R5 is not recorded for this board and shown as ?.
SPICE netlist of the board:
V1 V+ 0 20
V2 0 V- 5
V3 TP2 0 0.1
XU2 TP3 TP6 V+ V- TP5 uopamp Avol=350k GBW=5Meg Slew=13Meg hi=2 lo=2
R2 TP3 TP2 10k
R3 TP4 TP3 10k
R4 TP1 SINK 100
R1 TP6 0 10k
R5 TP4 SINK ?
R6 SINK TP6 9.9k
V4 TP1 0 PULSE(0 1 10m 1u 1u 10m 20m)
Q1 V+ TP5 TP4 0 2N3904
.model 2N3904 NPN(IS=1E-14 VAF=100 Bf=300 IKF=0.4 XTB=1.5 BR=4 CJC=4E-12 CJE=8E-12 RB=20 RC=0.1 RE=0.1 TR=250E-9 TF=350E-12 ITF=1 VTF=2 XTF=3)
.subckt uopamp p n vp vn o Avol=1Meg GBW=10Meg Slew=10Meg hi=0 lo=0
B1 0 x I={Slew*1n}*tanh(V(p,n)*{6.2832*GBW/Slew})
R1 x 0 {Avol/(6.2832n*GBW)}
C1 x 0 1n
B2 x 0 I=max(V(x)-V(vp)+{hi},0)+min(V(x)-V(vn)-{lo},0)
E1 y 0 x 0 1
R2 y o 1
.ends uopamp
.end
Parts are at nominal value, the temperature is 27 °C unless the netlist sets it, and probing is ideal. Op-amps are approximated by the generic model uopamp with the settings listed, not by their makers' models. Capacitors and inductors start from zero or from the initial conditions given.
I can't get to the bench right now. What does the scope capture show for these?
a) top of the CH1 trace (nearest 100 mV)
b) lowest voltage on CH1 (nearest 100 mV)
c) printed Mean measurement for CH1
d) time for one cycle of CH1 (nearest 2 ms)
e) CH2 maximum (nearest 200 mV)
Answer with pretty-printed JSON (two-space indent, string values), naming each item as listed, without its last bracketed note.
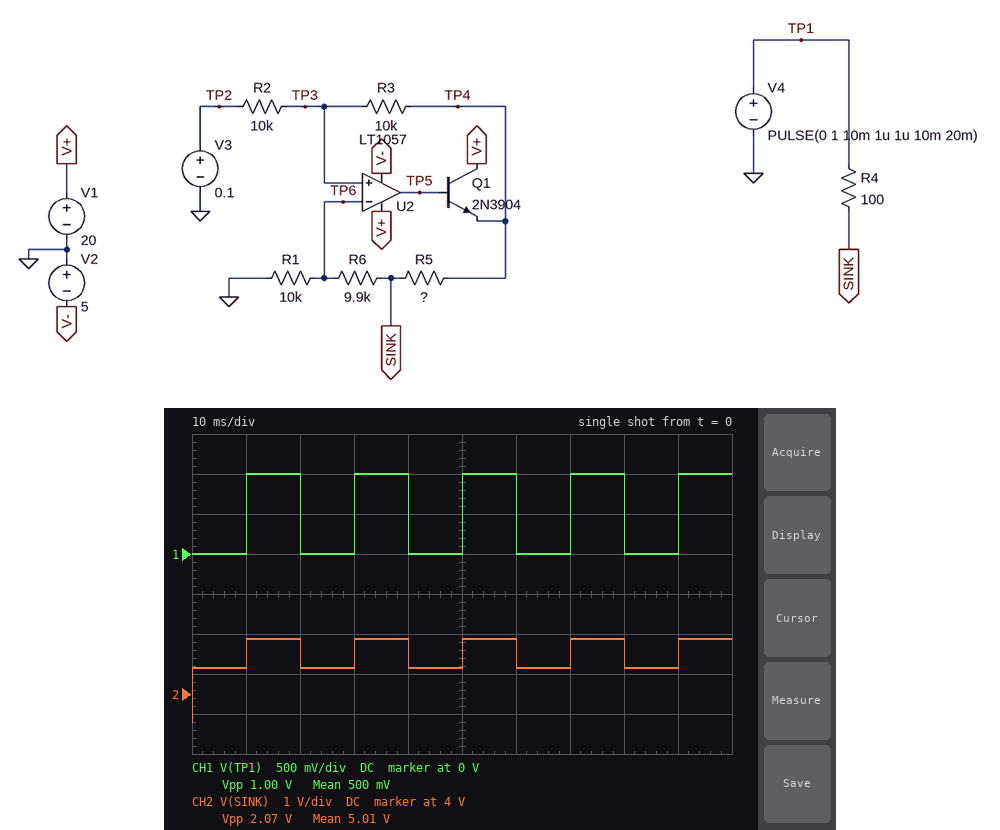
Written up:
{
  "top of the CH1 trace": "1.0 V",
  "lowest voltage on CH1": "0 V",
  "printed Mean measurement for CH1": "500 mV",
  "time for one cycle of CH1": "20 ms",
  "CH2 maximum": "5.4 V"
}
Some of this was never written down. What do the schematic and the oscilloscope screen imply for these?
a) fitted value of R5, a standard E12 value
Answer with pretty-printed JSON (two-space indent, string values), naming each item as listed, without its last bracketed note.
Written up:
{
  "fitted value of R5, a standard E12 value": "270 Ω"
}
